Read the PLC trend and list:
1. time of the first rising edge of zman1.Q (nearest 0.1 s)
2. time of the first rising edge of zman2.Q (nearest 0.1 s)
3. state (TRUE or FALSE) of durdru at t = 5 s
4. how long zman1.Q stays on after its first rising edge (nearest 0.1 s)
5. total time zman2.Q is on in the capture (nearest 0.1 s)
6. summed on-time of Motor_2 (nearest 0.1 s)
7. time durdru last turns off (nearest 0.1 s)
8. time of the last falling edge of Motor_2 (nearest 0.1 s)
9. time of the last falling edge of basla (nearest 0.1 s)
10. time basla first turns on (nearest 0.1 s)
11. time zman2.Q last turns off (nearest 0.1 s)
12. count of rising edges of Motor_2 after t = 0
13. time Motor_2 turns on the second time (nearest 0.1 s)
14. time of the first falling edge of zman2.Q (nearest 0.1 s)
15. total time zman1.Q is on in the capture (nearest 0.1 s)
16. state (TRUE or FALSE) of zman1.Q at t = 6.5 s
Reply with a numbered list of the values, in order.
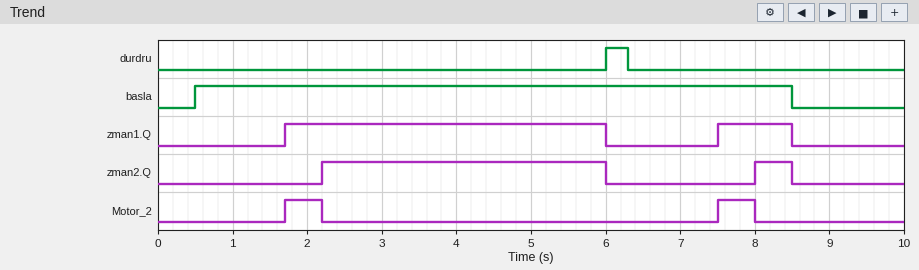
1. 1.7 s
2. 2.2 s
3. FALSE
4. 4.3 s
5. 4.3 s
6. 1.0 s
7. 6.3 s
8. 8.0 s
9. 8.5 s
10. 0.5 s
11. 8.5 s
12. 2
13. 7.5 s
14. 6.0 s
15. 5.3 s
16. FALSE
